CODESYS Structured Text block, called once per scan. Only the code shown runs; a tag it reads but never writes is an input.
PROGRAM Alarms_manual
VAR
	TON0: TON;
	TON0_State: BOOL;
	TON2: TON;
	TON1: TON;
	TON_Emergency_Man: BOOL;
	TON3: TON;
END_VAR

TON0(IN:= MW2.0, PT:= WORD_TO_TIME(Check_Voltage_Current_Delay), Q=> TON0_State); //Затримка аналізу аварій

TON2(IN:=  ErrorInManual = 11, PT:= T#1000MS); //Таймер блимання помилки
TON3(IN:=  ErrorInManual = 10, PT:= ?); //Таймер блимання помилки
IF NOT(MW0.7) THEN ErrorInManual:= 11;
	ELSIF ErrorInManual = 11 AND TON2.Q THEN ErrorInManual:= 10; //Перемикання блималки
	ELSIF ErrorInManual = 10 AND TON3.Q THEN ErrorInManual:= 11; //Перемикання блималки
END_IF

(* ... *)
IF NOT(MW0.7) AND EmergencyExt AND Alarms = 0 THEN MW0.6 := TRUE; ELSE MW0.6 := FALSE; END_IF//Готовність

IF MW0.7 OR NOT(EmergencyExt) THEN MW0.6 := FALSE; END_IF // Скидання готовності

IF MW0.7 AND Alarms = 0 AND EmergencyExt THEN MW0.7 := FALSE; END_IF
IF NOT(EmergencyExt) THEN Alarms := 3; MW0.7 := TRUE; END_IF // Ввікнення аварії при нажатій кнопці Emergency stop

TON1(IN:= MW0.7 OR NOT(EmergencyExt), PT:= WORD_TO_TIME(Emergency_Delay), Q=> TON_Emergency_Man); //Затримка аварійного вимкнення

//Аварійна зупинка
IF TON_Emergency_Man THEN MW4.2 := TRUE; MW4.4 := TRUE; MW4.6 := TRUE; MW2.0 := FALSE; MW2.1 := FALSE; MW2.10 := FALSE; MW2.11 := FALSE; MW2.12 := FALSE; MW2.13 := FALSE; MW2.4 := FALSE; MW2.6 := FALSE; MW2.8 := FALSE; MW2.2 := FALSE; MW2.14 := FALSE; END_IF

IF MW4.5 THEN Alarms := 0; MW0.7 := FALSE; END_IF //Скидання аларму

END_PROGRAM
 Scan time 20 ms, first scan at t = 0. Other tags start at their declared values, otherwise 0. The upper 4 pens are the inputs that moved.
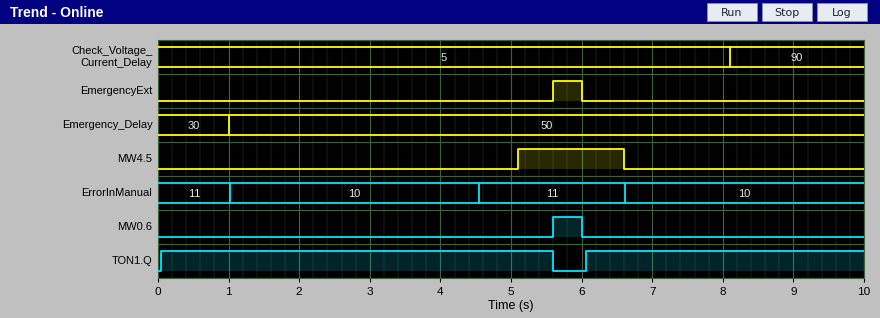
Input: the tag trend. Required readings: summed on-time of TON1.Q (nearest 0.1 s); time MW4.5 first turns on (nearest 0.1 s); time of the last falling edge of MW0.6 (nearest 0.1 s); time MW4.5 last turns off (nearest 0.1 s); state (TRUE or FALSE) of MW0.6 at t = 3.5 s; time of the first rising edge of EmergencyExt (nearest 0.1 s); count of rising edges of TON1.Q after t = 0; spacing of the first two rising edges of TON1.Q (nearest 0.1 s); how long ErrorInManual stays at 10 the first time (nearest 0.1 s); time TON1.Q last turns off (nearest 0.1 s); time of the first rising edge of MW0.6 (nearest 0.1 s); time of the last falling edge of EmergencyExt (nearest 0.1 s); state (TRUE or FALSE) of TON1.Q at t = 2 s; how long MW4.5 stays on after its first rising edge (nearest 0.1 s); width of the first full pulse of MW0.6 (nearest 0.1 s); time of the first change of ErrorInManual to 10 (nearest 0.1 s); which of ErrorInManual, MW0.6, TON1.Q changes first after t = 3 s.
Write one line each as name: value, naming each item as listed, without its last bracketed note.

summed on-time of TON1.Q: 9.5 s
time MW4.5 first turns on: 5.1 s
time of the last falling edge of MW0.6: 6.0 s
time MW4.5 last turns off: 6.6 s
state (TRUE or FALSE) of MW0.6 at t = 3.5 s: FALSE
time of the first rising edge of EmergencyExt: 5.6 s
count of rising edges of TON1.Q after t = 0: 2
spacing of the first two rising edges of TON1.Q: 6.0 s
how long ErrorInManual stays at 10 the first time: 3.5 s
time TON1.Q last turns off: 5.6 s
time of the first rising edge of MW0.6: 5.6 s
time of the last falling edge of EmergencyExt: 6.0 s
state (TRUE or FALSE) of TON1.Q at t = 2 s: TRUE
how long MW4.5 stays on after its first rising edge: 1.5 s
width of the first full pulse of MW0.6: 0.4 s
time of the first change of ErrorInManual to 10: 1.0 s
which of ErrorInManual, MW0.6, TON1.Q changes first after t = 3 s: ErrorInManual
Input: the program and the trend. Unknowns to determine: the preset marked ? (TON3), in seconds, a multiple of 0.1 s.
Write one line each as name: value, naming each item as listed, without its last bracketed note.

the preset marked ? (TON3), in seconds, a multiple of 0.1 s: 3.5 s
